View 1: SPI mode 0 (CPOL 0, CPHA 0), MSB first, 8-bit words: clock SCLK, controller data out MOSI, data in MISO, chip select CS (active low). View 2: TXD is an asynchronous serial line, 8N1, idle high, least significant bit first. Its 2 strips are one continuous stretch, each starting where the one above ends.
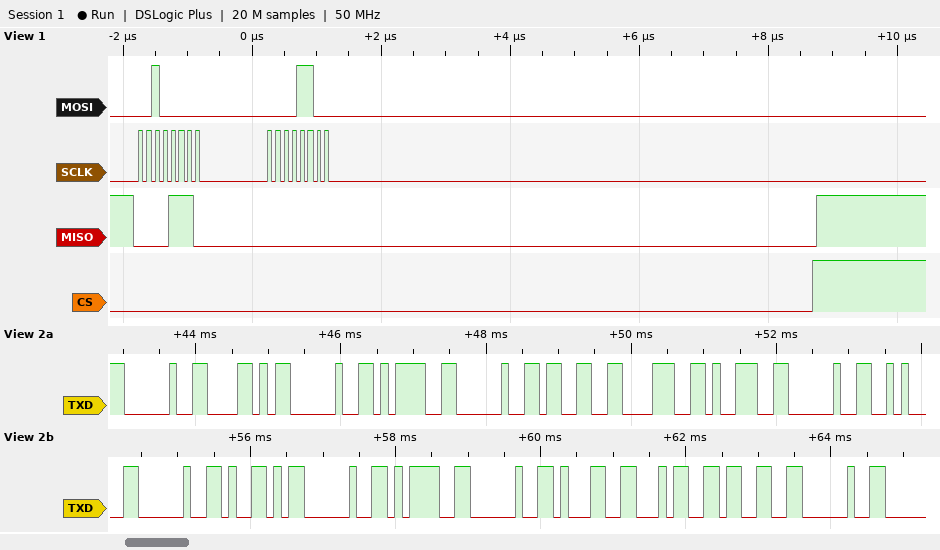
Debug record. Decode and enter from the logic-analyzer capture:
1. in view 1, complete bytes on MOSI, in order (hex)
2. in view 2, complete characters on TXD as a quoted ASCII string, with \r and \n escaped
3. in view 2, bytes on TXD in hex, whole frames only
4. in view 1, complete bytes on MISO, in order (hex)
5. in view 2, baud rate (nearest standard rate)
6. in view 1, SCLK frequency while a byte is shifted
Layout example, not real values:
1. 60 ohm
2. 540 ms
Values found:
1. 0x20 0x0C
2. " X = 389 \n Y = 143 "
3. 0x20 0x58 0x20 0x3D 0x20 0x33 0x38 0x39 0x20 0x0A 0x20 0x59 0x20 0x3D 0x20 0x31 0x34 0x33 0x20
4. 0x0E 0x00
5. 9600 baud
6. 8 MHz
